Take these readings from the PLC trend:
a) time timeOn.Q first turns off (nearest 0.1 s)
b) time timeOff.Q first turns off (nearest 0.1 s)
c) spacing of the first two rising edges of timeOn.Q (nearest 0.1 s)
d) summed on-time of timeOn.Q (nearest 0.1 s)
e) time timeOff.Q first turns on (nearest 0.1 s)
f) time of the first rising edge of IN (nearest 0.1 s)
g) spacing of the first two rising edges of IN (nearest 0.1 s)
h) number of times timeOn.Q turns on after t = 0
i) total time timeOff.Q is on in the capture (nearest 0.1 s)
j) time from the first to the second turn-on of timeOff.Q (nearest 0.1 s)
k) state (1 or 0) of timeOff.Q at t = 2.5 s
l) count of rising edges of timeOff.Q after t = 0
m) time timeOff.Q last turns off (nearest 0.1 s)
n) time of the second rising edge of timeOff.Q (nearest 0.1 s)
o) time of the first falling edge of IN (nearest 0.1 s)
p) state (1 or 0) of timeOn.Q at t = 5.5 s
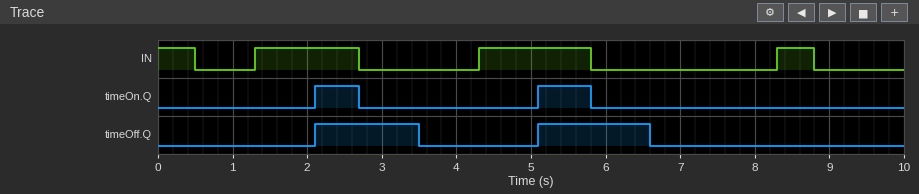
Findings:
2.7 s
3.5 s
3.0 s
1.3 s
2.1 s
1.3 s
3.0 s
2
2.9 s
3.0 s
1
2
6.6 s
5.1 s
0.5 s
1
